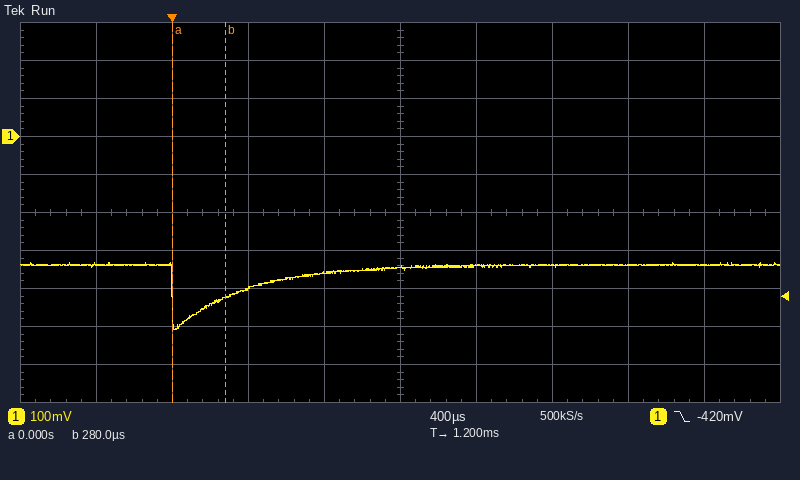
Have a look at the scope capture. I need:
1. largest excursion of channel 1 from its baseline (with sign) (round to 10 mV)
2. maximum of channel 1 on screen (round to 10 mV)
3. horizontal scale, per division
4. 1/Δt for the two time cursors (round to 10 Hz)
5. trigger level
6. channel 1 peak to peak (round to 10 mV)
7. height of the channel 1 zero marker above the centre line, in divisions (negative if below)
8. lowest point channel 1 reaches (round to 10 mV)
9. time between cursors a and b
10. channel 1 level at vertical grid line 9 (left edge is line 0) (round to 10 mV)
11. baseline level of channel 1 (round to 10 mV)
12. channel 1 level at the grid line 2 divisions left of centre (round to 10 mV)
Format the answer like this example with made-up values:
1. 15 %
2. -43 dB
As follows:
1. -170 mV
2. -330 mV
3. 400 µs
4. 3.57 kHz
5. -420 mV
6. 180 mV
7. +2.0 div
8. -510 mV
9. 280 µs
10. -340 mV
11. -340 mV
12. -400 mV
